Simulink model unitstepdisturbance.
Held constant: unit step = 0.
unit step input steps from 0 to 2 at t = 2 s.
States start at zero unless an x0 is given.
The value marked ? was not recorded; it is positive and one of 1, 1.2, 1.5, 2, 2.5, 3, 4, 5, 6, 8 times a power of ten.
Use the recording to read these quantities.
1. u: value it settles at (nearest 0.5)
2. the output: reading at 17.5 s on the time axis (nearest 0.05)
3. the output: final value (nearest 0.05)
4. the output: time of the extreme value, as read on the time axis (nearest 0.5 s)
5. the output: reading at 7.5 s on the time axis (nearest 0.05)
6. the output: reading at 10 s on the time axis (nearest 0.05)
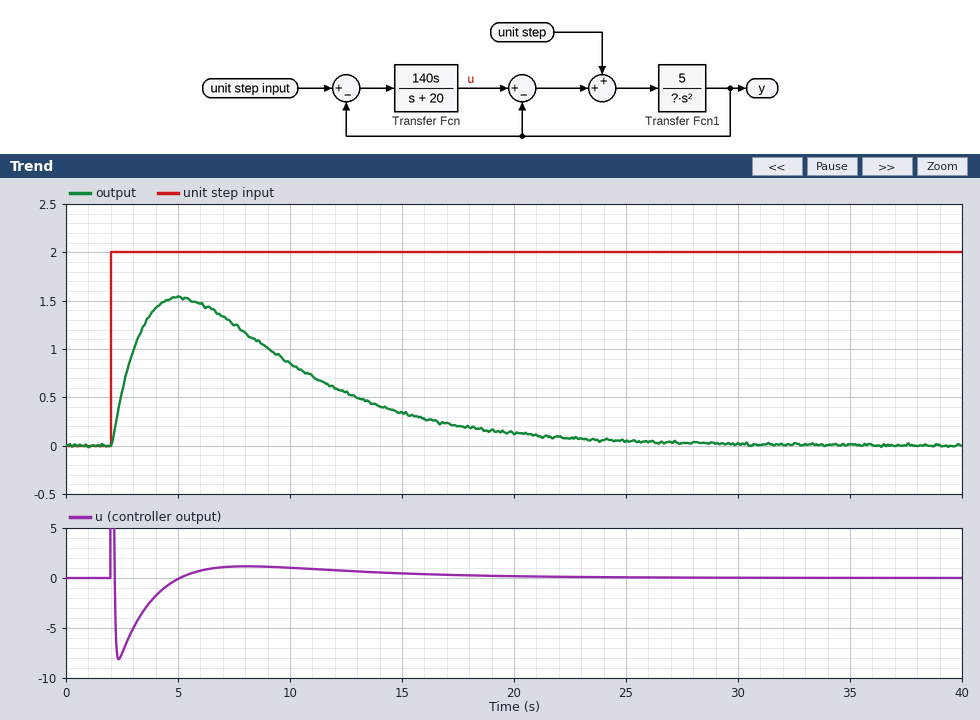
0.0
0.20
0.00
5.0 s
1.25
0.85
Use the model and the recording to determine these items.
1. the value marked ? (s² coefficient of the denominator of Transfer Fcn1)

50
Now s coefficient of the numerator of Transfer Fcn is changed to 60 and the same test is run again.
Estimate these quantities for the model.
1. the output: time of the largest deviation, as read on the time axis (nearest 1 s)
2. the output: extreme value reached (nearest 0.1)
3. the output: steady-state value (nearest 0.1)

6 s
1.1
0.0
